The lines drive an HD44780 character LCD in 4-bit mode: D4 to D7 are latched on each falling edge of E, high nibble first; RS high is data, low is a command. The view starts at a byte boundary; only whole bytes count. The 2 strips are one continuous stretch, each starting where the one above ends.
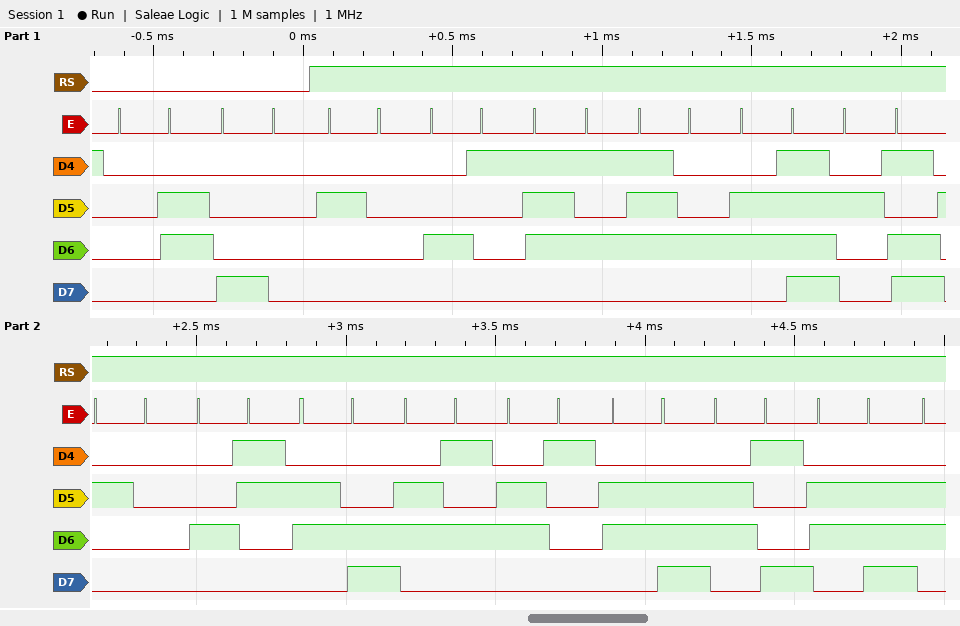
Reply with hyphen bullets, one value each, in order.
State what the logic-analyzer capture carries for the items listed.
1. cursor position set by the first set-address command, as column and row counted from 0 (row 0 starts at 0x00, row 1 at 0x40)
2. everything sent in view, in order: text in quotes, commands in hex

- column 0, row 0
- 0x06 0x80 " Auto- Cleanin"
